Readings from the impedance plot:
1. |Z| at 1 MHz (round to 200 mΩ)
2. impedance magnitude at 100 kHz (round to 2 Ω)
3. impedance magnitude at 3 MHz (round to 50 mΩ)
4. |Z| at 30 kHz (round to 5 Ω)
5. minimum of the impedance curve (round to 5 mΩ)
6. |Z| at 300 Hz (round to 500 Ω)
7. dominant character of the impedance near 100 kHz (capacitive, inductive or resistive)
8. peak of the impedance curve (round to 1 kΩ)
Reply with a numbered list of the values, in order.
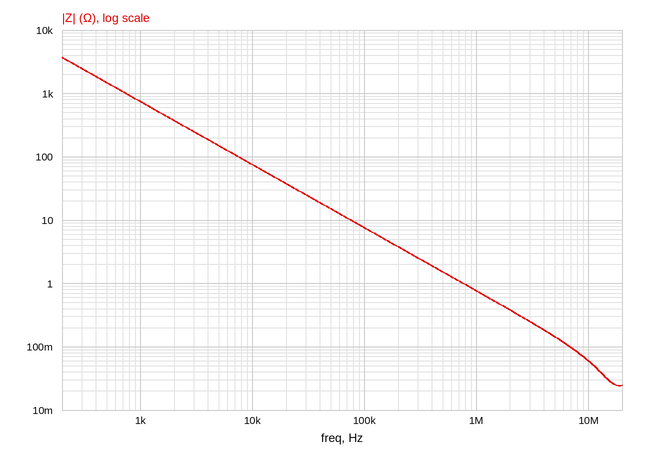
1. 800 mΩ
2. 8 Ω
3. 250 mΩ
4. 25 Ω
5. 25 mΩ
6. 2.5 kΩ
7. capacitive
8. 4 kΩ
